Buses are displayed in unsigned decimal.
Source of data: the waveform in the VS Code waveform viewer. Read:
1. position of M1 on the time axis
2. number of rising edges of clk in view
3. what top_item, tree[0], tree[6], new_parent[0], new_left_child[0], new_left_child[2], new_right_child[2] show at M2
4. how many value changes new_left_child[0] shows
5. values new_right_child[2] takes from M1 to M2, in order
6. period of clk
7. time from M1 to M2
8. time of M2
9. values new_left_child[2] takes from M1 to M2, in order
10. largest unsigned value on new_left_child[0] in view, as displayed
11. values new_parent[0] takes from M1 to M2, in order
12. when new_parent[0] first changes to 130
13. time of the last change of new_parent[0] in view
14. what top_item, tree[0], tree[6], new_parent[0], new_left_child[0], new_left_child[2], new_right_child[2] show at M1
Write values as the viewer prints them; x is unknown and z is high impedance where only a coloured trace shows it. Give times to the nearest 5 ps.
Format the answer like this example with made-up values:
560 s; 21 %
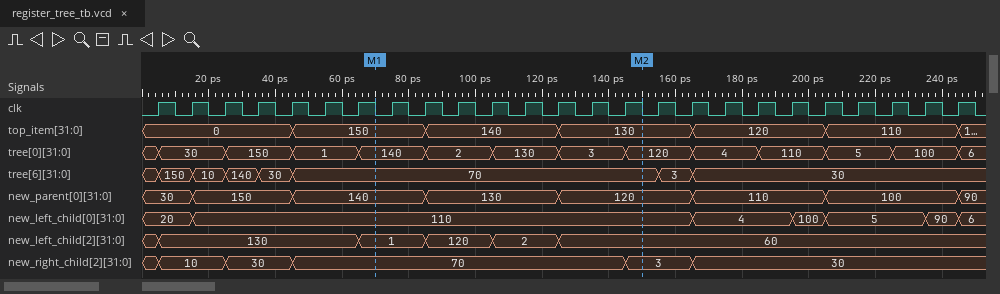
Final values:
70 ps; 25; top_item=130, tree[0]=120, tree[6]=70, new_parent[0]=120, new_left_child[0]=110, new_left_child[2]=60, new_right_child[2]=3; 6; 70, 3; 10 ps; 80 ps; 150 ps; 1, 120, 2, 60; 110; 140, 130, 120; 85 ps; 245 ps; top_item=150, tree[0]=140, tree[6]=70, new_parent[0]=140, new_left_child[0]=110, new_left_child[2]=1, new_right_child[2]=70
